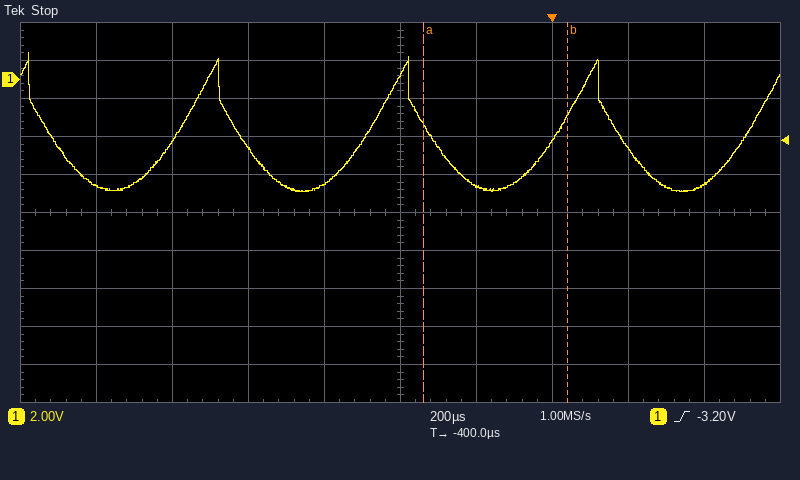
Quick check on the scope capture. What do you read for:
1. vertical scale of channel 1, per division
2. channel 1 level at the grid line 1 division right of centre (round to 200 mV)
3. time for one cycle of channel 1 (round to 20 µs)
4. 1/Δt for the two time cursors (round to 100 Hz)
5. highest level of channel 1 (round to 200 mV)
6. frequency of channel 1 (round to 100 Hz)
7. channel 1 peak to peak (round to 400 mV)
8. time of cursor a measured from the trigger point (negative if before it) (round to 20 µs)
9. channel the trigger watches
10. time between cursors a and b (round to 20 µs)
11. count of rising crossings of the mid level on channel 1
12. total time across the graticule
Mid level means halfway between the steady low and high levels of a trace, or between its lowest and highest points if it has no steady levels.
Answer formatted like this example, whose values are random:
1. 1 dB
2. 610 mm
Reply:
1. 2 V
2. -5.6 V
3. 500 µs
4. 2.6 kHz
5. 1.4 V
6. 2.0 kHz
7. 7.2 V
8. -340 µs
9. channel 1
10. 380 µs
11. 4
12. 2 ms
